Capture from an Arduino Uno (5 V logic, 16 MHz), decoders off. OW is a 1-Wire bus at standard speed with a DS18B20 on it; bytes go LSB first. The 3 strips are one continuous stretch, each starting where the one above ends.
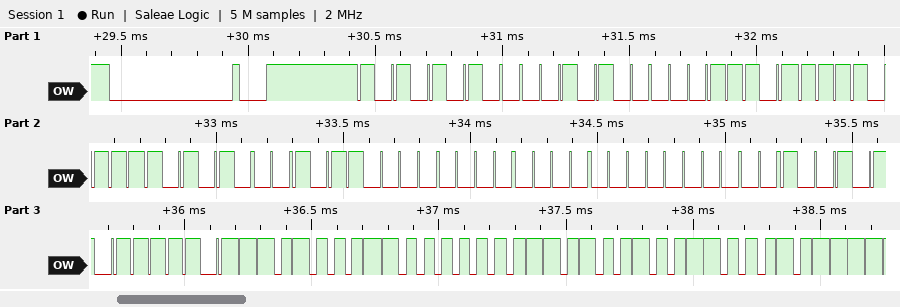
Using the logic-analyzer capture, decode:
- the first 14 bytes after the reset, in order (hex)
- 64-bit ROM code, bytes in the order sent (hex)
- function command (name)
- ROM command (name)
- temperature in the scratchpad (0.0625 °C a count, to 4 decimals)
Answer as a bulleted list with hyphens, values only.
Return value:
- 55 28 B8 EF 15 0D 00 00 A4 BE 8B 01 4B 46
- 28 B8 EF 15 0D 00 00 A4
- Read Scratchpad
- Match ROM
- 24.6875 °C
